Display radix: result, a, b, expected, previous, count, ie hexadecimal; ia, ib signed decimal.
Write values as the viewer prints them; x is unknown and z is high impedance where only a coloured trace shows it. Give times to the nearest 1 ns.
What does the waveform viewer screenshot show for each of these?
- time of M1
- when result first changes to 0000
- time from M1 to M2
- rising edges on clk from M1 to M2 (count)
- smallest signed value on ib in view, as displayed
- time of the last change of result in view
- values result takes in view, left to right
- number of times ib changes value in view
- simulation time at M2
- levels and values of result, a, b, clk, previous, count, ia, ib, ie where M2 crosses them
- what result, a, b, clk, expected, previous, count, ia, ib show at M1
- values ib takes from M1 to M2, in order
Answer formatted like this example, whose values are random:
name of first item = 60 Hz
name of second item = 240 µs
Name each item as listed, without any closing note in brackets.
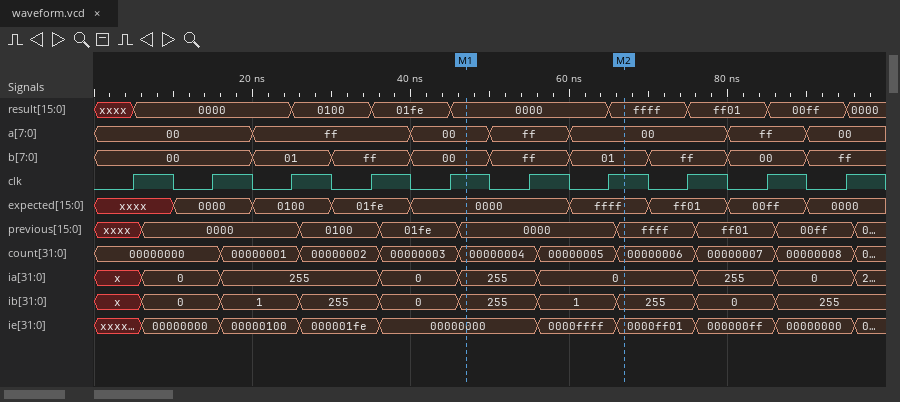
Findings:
time of M1 = 47 ns
when result first changes to 0000 = 5 ns
time from M1 to M2 = 20 ns
rising edges on clk from M1 to M2 = 2
smallest signed value on ib in view, as displayed = 0
time of the last change of result in view = 95 ns
values result takes in view, left to right = xxxx, 0000, 0100, 01fe, 0000, ffff, ff01, 00ff, 0000
number of times ib changes value in view = 9
simulation time at M2 = 67 ns
levels and values of result, a, b, clk, previous, count, ia, ib, ie where M2 crosses them = result=ffff, a=00, b=01, clk=1, previous=ffff, count=00000006, ia=0, ib=255, ie=0000ff01
what result, a, b, clk, expected, previous, count, ia, ib show at M1 = result=0000, a=00, b=00, clk=1, expected=0000, previous=0000, count=00000004, ia=255, ib=255
values ib takes from M1 to M2, in order = 255, 1, 255
